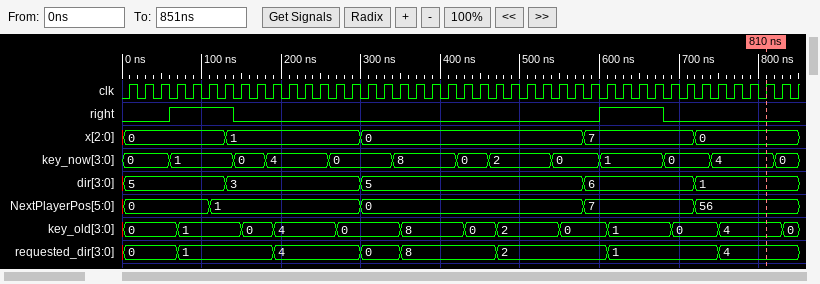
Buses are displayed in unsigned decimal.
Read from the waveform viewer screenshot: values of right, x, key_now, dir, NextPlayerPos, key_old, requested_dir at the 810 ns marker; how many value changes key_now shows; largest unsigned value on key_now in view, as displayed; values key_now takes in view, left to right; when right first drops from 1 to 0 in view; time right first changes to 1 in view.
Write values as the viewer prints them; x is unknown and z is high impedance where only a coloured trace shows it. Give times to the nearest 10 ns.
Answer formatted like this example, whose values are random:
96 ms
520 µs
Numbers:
right=0, x=0, key_now=4, dir=1, NextPlayerPos=56, key_old=4, requested_dir=4
12
8
0, 1, 0, 4, 0, 8, 0, 2, 0, 1, 0, 4, 0
140 ns
60 ns
